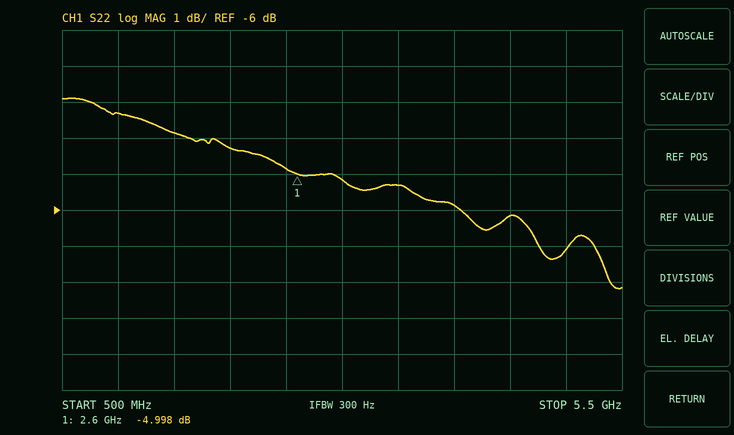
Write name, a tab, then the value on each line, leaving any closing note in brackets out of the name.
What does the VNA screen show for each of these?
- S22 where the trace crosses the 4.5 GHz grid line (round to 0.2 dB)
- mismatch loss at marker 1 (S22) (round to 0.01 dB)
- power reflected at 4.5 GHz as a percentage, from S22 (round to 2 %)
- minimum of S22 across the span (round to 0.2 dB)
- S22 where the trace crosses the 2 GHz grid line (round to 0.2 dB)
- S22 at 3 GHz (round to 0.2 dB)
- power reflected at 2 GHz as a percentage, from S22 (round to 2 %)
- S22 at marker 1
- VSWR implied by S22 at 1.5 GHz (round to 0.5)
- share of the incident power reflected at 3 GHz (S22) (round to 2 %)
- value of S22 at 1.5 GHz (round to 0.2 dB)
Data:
S22 where the trace crosses the 4.5 GHz grid line	-6.2 dB
mismatch loss at marker 1 (S22)	1.65 dB
power reflected at 4.5 GHz as a percentage, from S22	24 %
minimum of S22 across the span	-8.2 dB
S22 where the trace crosses the 2 GHz grid line	-4.2 dB
S22 at 3 GHz	-5.2 dB
power reflected at 2 GHz as a percentage, from S22	38 %
S22 at marker 1	-4.998 dB
VSWR implied by S22 at 1.5 GHz	4.5
share of the incident power reflected at 3 GHz (S22)	30 %
value of S22 at 1.5 GHz	-3.8 dB
